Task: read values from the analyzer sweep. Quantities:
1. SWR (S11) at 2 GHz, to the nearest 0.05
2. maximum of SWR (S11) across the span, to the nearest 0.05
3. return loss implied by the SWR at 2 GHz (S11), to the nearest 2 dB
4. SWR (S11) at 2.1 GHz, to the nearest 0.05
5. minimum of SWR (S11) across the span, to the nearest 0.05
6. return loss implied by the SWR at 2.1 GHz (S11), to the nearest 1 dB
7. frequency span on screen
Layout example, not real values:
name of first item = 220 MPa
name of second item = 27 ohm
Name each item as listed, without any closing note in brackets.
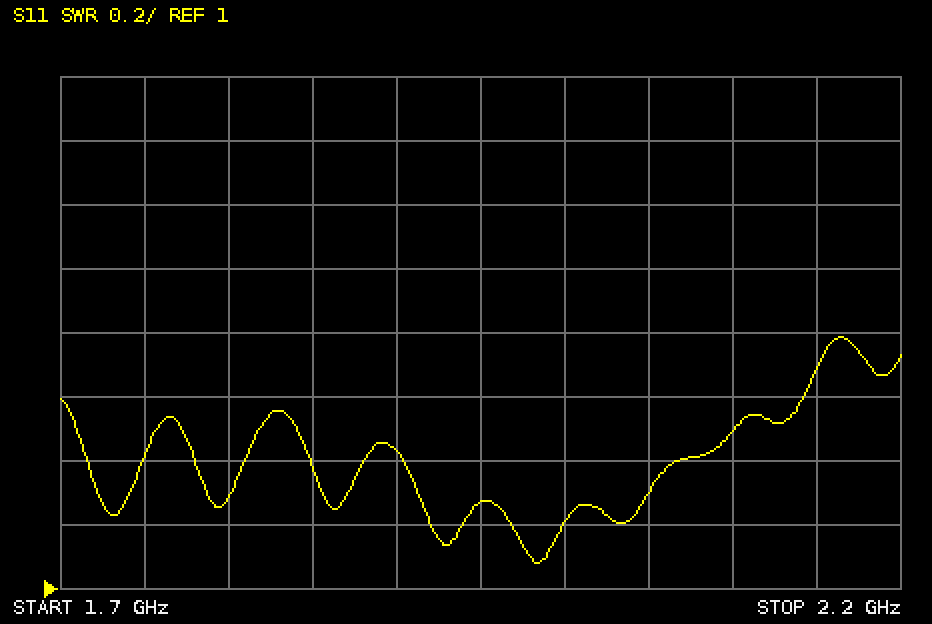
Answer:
SWR (S11) at 2 GHz, to the nearest 0.05 = 1.20
maximum of SWR (S11) across the span, to the nearest 0.05 = 1.80
return loss implied by the SWR at 2 GHz (S11), to the nearest 2 dB = 20 dB
SWR (S11) at 2.1 GHz, to the nearest 0.05 = 1.50
minimum of SWR (S11) across the span, to the nearest 0.05 = 1.10
return loss implied by the SWR at 2.1 GHz (S11), to the nearest 1 dB = 14 dB
frequency span on screen = 500 MHz
